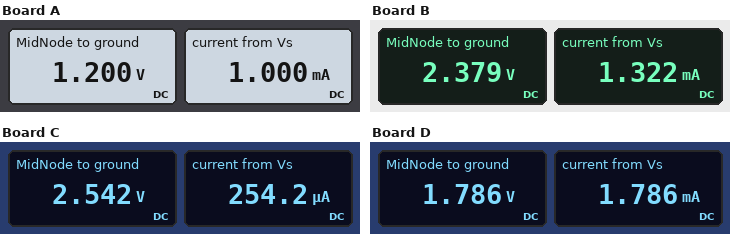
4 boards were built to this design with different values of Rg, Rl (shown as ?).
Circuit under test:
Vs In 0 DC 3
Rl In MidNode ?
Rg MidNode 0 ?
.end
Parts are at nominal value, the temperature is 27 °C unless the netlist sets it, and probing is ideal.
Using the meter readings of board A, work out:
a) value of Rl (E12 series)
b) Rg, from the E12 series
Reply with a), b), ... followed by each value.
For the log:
a) 1.8 kΩ
b) 1.2 kΩ
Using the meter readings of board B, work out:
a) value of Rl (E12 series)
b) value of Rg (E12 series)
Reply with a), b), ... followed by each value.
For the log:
a) 470 Ω
b) 1.8 kΩ
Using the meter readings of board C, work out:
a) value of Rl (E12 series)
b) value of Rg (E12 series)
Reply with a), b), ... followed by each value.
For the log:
a) 1.8 kΩ
b) 10 kΩ
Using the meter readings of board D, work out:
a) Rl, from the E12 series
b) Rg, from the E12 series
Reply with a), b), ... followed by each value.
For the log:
a) 680 Ω
b) 1 kΩ
